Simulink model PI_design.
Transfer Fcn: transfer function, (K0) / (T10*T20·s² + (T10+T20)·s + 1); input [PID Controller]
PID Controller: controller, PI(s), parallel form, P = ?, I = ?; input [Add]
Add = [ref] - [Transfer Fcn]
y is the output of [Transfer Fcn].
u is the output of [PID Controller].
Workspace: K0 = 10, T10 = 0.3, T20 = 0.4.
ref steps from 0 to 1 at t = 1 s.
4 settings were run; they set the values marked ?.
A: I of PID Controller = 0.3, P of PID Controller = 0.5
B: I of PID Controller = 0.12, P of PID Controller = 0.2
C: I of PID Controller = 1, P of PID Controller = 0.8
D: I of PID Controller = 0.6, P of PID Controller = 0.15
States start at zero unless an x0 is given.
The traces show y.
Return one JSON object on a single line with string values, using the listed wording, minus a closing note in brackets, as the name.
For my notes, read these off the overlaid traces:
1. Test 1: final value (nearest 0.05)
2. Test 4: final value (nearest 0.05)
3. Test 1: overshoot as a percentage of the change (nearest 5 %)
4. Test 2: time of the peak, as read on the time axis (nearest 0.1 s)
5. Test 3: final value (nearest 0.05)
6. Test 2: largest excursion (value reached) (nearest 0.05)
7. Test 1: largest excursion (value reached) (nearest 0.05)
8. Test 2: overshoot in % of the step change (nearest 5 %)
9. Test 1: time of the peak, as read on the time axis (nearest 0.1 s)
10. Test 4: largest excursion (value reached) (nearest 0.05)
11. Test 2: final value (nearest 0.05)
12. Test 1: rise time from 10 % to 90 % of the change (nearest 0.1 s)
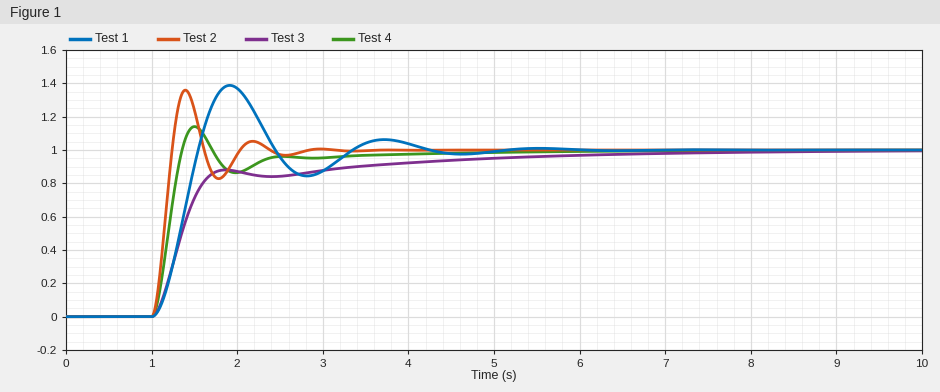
{"Test 1: final value": "1.00", "Test 4: final value": "1.00", "Test 1: overshoot as a percentage of the change": "40 %", "Test 2: time of the peak, as read on the time axis": "1.4 s", "Test 3: final value": "1.00", "Test 2: largest excursion (value reached)": "1.35", "Test 1: largest excursion (value reached)": "1.40", "Test 2: overshoot in % of the step change": "35 %", "Test 1: time of the peak, as read on the time axis": "1.9 s", "Test 4: largest excursion (value reached)": "1.15", "Test 2: final value": "1.00", "Test 1: rise time from 10 % to 90 % of the change": "0.4 s"}
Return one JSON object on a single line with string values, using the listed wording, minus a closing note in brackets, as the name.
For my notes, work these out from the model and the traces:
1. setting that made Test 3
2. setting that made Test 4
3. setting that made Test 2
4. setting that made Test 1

{"setting that made Test 3": "B", "setting that made Test 4": "A", "setting that made Test 2": "C", "setting that made Test 1": "D"}
